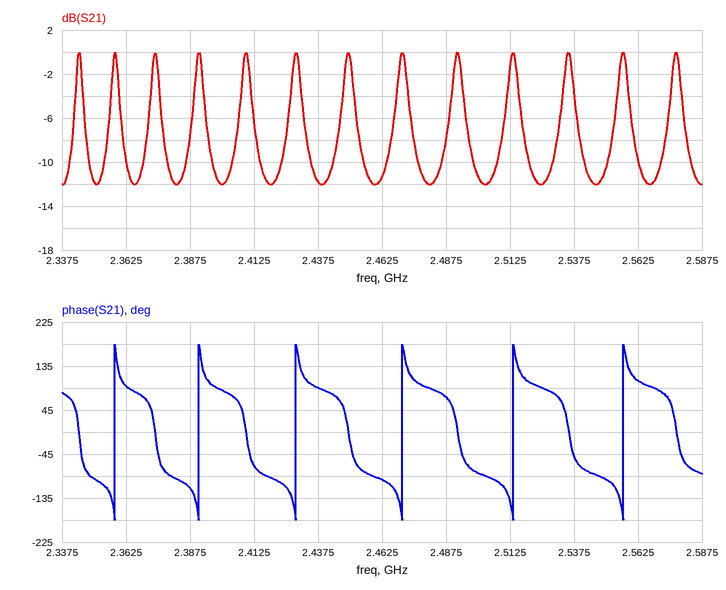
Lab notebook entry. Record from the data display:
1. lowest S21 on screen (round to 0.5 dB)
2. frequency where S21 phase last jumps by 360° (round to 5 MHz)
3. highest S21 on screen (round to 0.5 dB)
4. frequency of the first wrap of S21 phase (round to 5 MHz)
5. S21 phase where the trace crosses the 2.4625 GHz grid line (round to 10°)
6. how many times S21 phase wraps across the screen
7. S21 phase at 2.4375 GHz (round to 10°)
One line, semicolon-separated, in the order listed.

-12.0 dB; 2.555 GHz; 0.0 dB; 2.360 GHz; -100°; 6; 90°
